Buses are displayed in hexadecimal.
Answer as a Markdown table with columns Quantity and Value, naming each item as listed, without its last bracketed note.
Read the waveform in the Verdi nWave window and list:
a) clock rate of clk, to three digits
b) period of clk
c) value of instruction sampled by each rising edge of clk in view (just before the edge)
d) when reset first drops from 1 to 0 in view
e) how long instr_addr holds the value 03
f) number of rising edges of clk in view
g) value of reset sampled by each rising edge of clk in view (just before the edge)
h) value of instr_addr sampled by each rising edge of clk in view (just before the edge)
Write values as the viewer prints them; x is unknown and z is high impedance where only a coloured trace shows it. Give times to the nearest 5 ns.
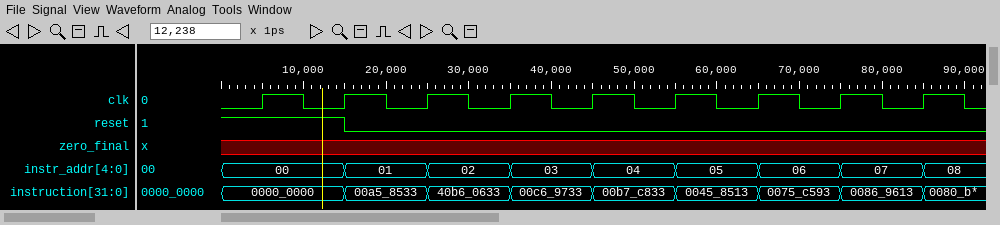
| Quantity | Value |
|---|---|
| clock rate of clk, to three digits | 100 MHz |
| period of clk | 10 ns |
| value of instruction sampled by each rising edge of clk in view | 0000_0000, 0000_0000, 00a5_8533, 40b6_0633, 00c6_9733, 00b7_c833, 0045_8513, 0075_c593, 0086_9613 |
| when reset first drops from 1 to 0 in view | 15 ns |
| how long instr_addr holds the value 03 | 10 ns |
| number of rising edges of clk in view | 9 |
| value of reset sampled by each rising edge of clk in view | 1 1 0 0 0 0 0 0 0 |
| value of instr_addr sampled by each rising edge of clk in view | 00, 00, 01, 02, 03, 04, 05, 06, 07 |
